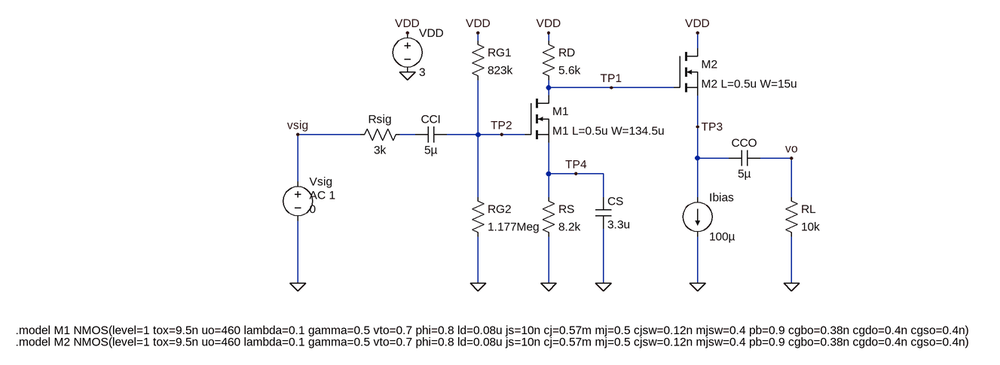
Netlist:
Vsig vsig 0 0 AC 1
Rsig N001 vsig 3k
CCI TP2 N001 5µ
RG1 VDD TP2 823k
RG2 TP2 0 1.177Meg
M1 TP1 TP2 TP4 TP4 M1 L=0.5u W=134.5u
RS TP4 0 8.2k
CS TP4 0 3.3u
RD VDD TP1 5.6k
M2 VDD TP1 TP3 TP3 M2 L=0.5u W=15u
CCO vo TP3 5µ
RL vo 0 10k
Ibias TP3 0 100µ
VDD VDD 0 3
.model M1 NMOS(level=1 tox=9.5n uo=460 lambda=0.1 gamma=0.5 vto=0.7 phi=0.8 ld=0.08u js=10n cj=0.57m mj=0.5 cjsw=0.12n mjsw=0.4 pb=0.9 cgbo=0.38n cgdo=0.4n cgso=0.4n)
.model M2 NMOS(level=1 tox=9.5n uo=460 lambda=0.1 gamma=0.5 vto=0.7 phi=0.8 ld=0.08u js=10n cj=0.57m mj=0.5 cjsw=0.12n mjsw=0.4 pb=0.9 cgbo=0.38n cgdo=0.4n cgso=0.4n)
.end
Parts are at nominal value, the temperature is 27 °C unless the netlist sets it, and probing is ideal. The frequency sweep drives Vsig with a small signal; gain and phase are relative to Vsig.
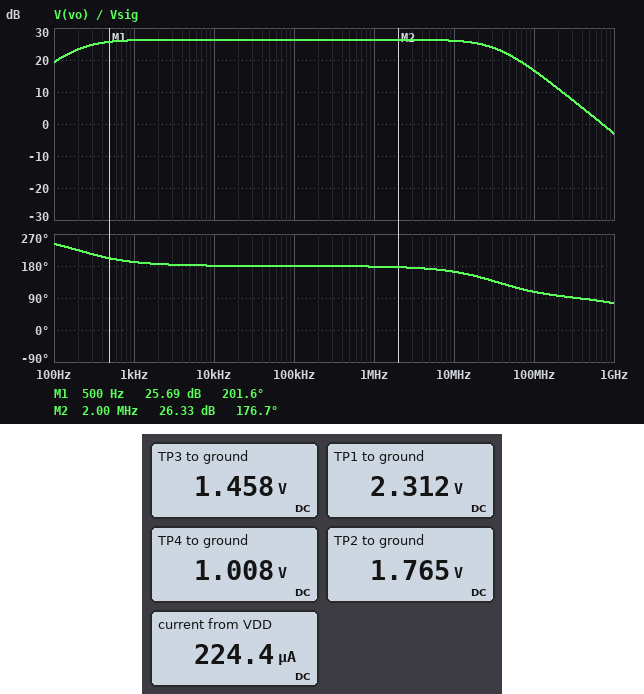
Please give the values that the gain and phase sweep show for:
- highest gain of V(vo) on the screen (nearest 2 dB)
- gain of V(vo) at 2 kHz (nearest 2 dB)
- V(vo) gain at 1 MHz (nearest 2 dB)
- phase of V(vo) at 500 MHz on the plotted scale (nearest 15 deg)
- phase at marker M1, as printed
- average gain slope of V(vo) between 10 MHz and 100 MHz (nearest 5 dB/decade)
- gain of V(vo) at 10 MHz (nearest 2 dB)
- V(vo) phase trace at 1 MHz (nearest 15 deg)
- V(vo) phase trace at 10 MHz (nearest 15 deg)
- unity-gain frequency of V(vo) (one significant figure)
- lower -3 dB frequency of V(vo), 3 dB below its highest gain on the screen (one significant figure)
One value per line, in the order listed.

26 dB
26 dB
26 dB
90 deg
201.6 deg
-10 dB/decade
26 dB
180 deg
165 deg
700 MHz
200 Hz
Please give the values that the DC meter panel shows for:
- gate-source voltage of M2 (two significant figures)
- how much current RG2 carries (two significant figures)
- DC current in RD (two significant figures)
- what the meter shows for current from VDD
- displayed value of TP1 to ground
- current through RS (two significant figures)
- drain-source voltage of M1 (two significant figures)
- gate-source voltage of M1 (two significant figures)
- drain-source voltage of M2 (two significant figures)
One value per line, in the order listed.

850 mV
1.5 µA
120 µA
224.4 µA
2.312 V
120 µA
1.3 V
760 mV
1.5 V
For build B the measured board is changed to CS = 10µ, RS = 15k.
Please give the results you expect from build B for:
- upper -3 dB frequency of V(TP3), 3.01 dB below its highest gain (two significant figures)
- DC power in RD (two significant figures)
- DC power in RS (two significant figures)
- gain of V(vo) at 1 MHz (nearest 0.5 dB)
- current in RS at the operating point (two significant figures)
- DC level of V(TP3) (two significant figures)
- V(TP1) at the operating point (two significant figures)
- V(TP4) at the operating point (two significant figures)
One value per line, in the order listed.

42 MHz
26 µW
70 µW
24.0 dB
68 µA
1.8 V
2.6 V
1.0 V
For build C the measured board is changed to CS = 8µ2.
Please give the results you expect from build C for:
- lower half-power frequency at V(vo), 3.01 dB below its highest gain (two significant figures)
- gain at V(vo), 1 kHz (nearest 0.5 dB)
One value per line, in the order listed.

81 Hz
26.5 dB
